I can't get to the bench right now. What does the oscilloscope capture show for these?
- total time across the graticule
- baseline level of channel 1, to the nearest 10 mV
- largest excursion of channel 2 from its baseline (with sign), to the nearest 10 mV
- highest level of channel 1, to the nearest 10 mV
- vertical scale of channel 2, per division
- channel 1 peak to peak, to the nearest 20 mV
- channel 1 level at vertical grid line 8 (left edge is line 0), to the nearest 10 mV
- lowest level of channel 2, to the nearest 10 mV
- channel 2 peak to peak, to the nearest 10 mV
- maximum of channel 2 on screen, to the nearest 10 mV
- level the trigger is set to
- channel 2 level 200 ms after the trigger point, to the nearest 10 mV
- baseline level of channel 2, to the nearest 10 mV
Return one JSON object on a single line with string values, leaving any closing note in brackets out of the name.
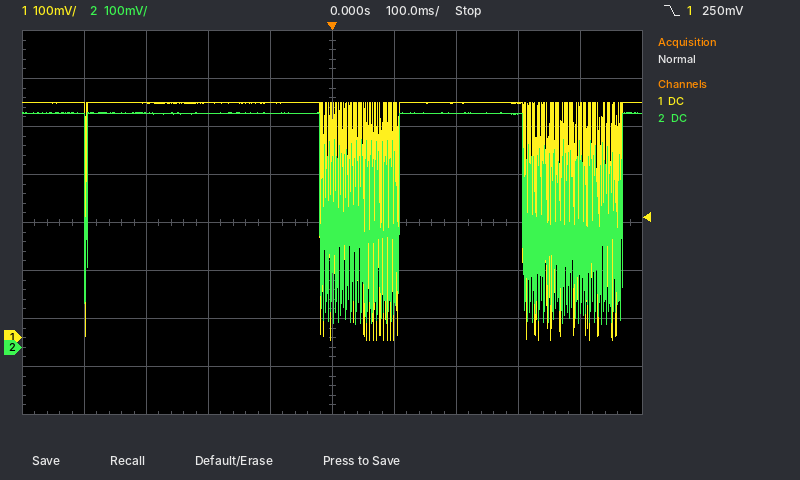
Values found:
{"total time across the graticule": "1 s", "baseline level of channel 1, to the nearest 10 mV": "490 mV", "largest excursion of channel 2 from its baseline (with sign), to the nearest 10 mV": "-440 mV", "highest level of channel 1, to the nearest 10 mV": "490 mV", "vertical scale of channel 2, per division": "100 mV", "channel 1 peak to peak, to the nearest 20 mV": "500 mV", "channel 1 level at vertical grid line 8 (left edge is line 0), to the nearest 10 mV": "490 mV", "lowest level of channel 2, to the nearest 10 mV": "50 mV", "channel 2 peak to peak, to the nearest 10 mV": "440 mV", "maximum of channel 2 on screen, to the nearest 10 mV": "490 mV", "level the trigger is set to": "250 mV", "channel 2 level 200 ms after the trigger point, to the nearest 10 mV": "490 mV", "baseline level of channel 2, to the nearest 10 mV": "490 mV"}
